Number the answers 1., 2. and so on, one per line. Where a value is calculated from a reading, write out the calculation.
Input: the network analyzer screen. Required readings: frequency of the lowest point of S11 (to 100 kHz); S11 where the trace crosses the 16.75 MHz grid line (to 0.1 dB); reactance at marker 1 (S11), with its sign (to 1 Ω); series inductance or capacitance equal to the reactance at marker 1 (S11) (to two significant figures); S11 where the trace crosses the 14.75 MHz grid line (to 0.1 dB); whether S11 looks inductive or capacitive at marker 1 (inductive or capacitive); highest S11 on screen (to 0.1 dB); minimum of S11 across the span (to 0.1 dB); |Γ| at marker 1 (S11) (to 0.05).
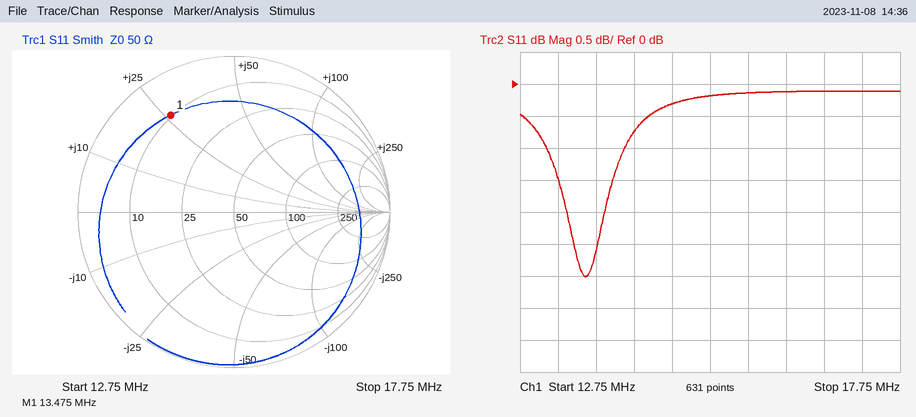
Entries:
1. 13.6 MHz
2. -0.1 dB
3. +26 Ω
4. L = 26 Ω/(2π × 13.475 MHz) ≈ 307 nH, so 310 nH to two significant figures
5. -0.3 dB
6. inductive
7. -0.1 dB
8. -3.0 dB
9. 0.75
